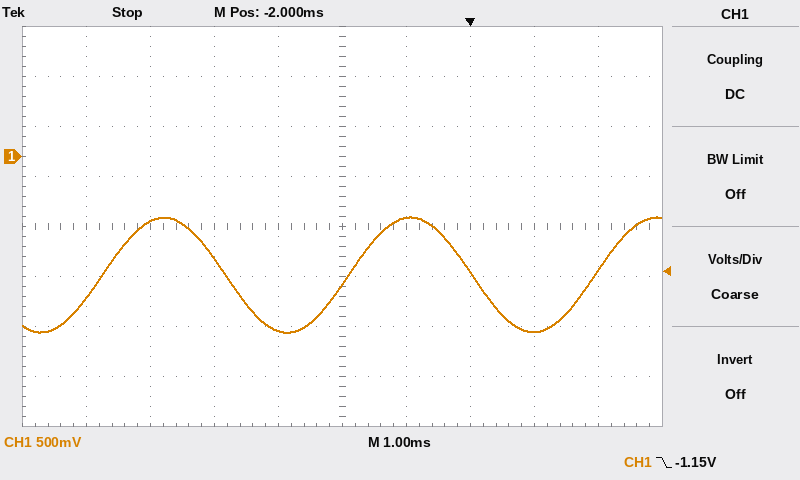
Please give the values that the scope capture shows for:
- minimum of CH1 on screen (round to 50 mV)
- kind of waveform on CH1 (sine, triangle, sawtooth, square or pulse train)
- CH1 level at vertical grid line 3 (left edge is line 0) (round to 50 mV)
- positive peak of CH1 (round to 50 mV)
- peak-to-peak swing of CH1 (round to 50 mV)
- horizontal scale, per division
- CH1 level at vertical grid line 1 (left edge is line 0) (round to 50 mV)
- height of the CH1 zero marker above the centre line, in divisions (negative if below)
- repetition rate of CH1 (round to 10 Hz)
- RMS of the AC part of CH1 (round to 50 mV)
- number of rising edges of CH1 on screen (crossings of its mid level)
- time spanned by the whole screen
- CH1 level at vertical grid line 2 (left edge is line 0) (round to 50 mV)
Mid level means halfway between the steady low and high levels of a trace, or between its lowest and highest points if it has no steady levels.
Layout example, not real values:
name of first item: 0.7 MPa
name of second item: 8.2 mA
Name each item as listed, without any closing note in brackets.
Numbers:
minimum of CH1 on screen: -1.75 V
kind of waveform on CH1: sine
CH1 level at vertical grid line 3 (left edge is line 0): -1.00 V
positive peak of CH1: -600 mV
peak-to-peak swing of CH1: 1.15 V
horizontal scale, per division: 1 ms
CH1 level at vertical grid line 1 (left edge is line 0): -1.40 V
height of the CH1 zero marker above the centre line, in divisions: +1.4 div
repetition rate of CH1: 260 Hz
RMS of the AC part of CH1: 400 mV
number of rising edges of CH1 on screen: 3
time spanned by the whole screen: 10 ms
CH1 level at vertical grid line 2 (left edge is line 0): -650 mV
